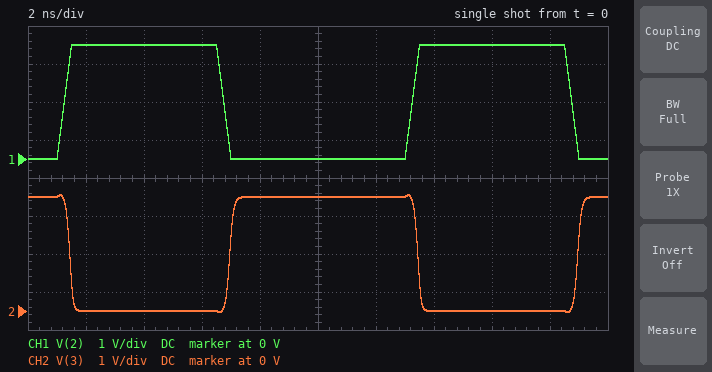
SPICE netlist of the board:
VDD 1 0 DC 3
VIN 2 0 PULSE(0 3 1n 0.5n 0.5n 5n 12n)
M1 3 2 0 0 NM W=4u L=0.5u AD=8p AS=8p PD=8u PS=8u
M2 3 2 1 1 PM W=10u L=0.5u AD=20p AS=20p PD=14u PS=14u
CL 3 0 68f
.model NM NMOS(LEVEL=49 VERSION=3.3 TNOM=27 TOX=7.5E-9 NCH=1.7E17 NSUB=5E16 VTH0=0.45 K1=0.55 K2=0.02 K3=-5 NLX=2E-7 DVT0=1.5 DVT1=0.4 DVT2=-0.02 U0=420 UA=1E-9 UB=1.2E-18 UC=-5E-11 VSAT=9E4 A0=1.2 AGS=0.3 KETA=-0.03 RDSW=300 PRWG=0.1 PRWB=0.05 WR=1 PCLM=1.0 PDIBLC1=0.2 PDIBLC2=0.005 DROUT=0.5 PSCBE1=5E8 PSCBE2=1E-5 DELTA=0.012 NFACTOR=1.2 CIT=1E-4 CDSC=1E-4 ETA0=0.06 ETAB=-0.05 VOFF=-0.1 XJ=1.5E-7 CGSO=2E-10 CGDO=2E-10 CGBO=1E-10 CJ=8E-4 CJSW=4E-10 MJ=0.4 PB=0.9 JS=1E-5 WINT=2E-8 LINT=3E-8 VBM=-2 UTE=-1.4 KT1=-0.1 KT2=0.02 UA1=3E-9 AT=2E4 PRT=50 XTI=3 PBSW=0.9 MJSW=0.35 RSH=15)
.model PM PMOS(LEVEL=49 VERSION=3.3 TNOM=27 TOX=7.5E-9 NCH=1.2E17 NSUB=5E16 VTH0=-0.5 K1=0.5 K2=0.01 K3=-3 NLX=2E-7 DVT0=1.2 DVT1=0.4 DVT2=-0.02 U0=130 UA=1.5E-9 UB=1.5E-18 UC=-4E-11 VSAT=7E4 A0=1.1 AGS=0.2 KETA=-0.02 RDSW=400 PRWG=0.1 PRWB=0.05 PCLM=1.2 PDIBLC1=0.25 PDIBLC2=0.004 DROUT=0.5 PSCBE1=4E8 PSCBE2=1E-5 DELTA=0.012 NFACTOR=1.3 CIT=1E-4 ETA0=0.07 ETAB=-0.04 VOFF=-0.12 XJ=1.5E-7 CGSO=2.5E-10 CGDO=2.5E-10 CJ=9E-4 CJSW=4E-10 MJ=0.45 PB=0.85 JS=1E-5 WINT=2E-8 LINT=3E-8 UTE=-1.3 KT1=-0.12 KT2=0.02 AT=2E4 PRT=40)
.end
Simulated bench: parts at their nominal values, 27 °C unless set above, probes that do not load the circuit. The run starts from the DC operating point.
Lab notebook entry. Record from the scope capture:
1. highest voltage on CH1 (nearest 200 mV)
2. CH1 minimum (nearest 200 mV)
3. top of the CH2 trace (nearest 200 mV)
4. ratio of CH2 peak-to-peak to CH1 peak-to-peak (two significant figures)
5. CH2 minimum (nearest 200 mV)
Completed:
3.0 V
0 V
3.0 V
1.0
0 V
